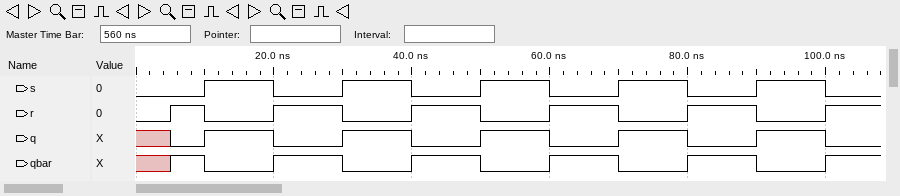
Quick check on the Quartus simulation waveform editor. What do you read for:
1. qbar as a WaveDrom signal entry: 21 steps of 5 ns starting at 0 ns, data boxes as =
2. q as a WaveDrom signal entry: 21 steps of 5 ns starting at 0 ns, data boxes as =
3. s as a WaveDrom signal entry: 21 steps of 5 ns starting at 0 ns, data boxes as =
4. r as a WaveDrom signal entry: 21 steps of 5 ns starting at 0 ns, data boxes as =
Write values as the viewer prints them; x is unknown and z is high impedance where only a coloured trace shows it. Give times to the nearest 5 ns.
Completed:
{name: 'qbar', wave: 'x10.1.0.1.0.1.0.1.0.1'}
{name: 'q', wave: 'x01.0.1.0.1.0.1.0.1.0'}
{name: 's', wave: '0.1.0.1.0.1.0.1.0.1.0'}
{name: 'r', wave: '010.1.0.1.0.1.0.1.0.1'}
